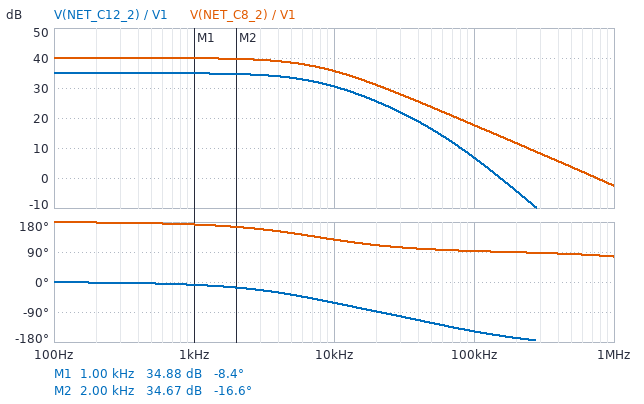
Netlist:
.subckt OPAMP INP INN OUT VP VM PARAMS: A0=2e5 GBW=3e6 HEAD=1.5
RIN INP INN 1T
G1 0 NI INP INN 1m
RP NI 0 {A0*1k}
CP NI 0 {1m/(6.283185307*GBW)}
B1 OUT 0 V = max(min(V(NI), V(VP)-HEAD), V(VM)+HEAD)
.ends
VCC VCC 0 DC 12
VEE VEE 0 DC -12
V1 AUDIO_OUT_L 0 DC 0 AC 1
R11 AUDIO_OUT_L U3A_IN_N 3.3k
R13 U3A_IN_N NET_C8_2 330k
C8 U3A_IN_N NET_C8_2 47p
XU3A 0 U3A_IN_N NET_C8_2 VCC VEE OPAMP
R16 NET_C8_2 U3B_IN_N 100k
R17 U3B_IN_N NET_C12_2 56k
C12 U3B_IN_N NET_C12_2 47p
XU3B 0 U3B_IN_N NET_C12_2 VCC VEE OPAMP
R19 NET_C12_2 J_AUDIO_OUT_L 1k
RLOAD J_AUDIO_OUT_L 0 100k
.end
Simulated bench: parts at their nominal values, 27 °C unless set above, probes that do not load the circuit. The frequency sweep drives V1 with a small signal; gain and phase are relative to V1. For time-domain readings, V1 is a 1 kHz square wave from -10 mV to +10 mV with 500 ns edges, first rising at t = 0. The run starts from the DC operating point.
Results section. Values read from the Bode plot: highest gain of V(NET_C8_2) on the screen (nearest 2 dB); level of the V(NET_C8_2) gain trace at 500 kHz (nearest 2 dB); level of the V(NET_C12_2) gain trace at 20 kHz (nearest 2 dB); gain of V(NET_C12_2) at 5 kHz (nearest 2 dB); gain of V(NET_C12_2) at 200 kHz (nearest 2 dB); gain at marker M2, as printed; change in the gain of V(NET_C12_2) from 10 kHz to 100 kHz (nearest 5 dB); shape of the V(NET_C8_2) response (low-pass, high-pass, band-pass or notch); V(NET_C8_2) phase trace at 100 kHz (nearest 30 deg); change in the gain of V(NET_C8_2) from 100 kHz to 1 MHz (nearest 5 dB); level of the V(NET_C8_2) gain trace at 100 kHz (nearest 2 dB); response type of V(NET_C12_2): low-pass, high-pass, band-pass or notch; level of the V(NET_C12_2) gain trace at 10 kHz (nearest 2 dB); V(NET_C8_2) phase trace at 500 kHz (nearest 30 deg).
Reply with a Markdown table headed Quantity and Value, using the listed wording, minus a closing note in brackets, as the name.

| Quantity | Value |
|---|---|
| highest gain of V(NET_C8_2) on the screen | 40 dB |
| level of the V(NET_C8_2) gain trace at 500 kHz | 4 dB |
| level of the V(NET_C12_2) gain trace at 20 kHz | 26 dB |
| gain of V(NET_C12_2) at 5 kHz | 34 dB |
| gain of V(NET_C12_2) at 200 kHz | -4 dB |
| gain at marker M2, as printed | 34.67 dB |
| change in the gain of V(NET_C12_2) from 10 kHz to 100 kHz | -25 dB |
| shape of the V(NET_C8_2) response | low-pass |
| V(NET_C8_2) phase trace at 100 kHz | 90 deg |
| change in the gain of V(NET_C8_2) from 100 kHz to 1 MHz | -20 dB |
| level of the V(NET_C8_2) gain trace at 100 kHz | 18 dB |
| response type of V(NET_C12_2): low-pass, high-pass, band-pass or notch | low-pass |
| level of the V(NET_C12_2) gain trace at 10 kHz | 30 dB |
| V(NET_C8_2) phase trace at 500 kHz | 90 deg |
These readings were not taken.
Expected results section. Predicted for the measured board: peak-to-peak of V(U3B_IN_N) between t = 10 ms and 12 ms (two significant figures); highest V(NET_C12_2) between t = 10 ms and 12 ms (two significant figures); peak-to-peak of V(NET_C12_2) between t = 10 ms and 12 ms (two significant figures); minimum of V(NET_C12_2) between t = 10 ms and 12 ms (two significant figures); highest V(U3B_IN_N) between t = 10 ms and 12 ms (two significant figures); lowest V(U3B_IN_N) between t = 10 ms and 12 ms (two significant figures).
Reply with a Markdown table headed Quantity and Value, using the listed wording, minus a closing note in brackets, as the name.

| Quantity | Value |
|---|---|
| peak-to-peak of V(U3B_IN_N) between t = 10 ms and 12 ms | 4.3 mV |
| highest V(NET_C12_2) between t = 10 ms and 12 ms | 560 mV |
| peak-to-peak of V(NET_C12_2) between t = 10 ms and 12 ms | 1.1 V |
| minimum of V(NET_C12_2) between t = 10 ms and 12 ms | -560 mV |
| highest V(U3B_IN_N) between t = 10 ms and 12 ms | 2.1 mV |
| lowest V(U3B_IN_N) between t = 10 ms and 12 ms | -2.1 mV |
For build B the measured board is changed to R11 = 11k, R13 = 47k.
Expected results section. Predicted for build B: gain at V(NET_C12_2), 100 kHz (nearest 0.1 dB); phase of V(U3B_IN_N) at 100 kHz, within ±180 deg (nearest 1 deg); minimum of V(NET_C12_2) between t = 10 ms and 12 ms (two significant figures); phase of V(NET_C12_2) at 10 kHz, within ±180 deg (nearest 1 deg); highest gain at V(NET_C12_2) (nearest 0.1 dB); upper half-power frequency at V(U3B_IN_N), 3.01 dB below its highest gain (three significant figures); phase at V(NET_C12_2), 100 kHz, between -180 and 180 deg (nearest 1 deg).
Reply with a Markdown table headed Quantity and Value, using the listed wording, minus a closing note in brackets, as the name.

| Quantity | Value |
|---|---|
| gain at V(NET_C12_2), 100 kHz | -3.5 dB |
| phase of V(U3B_IN_N) at 100 kHz, within ±180 deg | 150 deg |
| minimum of V(NET_C12_2) between t = 10 ms and 12 ms | -24 mV |
| phase of V(NET_C12_2) at 10 kHz, within ±180 deg | -19 deg |
| highest gain at V(NET_C12_2) | 7.6 dB |
| upper half-power frequency at V(U3B_IN_N), 3.01 dB below its highest gain | 150 kHz |
| phase at V(NET_C12_2), 100 kHz, between -180 and 180 deg | -120 deg |
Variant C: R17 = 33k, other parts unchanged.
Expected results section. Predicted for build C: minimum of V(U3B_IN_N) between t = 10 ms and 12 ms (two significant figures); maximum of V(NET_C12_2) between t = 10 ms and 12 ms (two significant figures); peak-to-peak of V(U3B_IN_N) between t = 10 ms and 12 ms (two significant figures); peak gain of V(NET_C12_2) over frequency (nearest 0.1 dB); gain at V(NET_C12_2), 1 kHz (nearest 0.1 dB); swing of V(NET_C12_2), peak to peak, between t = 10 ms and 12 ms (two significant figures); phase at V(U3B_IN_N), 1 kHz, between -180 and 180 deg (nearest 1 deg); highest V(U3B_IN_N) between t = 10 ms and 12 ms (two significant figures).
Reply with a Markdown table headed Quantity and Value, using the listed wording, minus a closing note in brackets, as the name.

| Quantity | Value |
|---|---|
| minimum of V(U3B_IN_N) between t = 10 ms and 12 ms | -1.4 mV |
| maximum of V(NET_C12_2) between t = 10 ms and 12 ms | 330 mV |
| peak-to-peak of V(U3B_IN_N) between t = 10 ms and 12 ms | 2.8 mV |
| peak gain of V(NET_C12_2) over frequency | 30.4 dB |
| gain at V(NET_C12_2), 1 kHz | 30.3 dB |
| swing of V(NET_C12_2), peak to peak, between t = 10 ms and 12 ms | 660 mV |
| phase at V(U3B_IN_N), 1 kHz, between -180 and 180 deg | -99 deg |
| highest V(U3B_IN_N) between t = 10 ms and 12 ms | 1.4 mV |
